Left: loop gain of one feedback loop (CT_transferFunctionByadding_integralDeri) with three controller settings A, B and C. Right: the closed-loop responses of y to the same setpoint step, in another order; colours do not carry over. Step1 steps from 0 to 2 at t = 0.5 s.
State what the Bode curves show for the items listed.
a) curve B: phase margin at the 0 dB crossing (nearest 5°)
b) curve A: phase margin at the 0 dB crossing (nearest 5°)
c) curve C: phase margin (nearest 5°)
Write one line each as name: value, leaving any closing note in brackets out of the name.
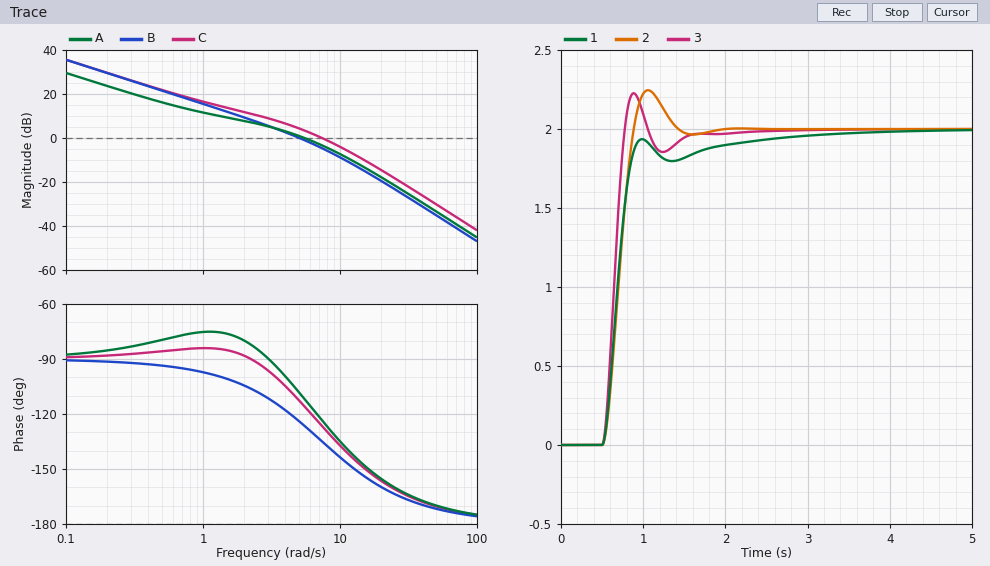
curve B: phase margin at the 0 dB crossing: 55°
curve A: phase margin at the 0 dB crossing: 70°
curve C: phase margin: 55°
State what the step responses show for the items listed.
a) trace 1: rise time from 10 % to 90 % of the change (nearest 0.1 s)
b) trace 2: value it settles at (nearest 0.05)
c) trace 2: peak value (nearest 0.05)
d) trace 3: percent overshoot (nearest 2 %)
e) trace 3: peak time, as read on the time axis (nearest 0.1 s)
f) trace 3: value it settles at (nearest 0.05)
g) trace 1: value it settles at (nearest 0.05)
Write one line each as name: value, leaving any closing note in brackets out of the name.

trace 1: rise time from 10 % to 90 % of the change: 0.3 s
trace 2: value it settles at: 2.00
trace 2: peak value: 2.25
trace 3: percent overshoot: 12 %
trace 3: peak time, as read on the time axis: 0.9 s
trace 3: value it settles at: 2.00
trace 1: value it settles at: 2.00
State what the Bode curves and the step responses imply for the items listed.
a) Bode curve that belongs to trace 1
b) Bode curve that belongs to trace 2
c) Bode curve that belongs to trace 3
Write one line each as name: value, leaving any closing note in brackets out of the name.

Bode curve that belongs to trace 1: A
Bode curve that belongs to trace 2: B
Bode curve that belongs to trace 3: C
